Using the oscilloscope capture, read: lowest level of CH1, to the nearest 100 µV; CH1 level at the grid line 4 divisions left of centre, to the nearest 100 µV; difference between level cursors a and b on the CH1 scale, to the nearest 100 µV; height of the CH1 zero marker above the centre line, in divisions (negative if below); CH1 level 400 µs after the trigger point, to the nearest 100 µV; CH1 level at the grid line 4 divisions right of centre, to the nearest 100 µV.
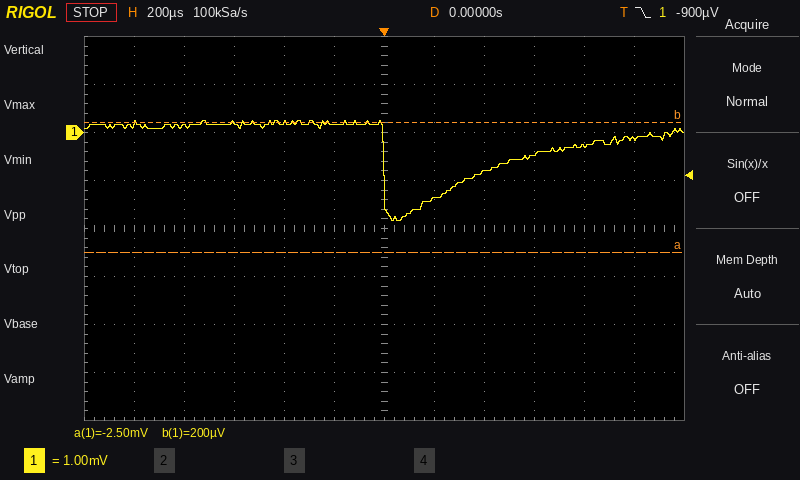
-1.8 mV
100 µV
2.7 mV
+2.0 div
-800 µV
-300 µV
